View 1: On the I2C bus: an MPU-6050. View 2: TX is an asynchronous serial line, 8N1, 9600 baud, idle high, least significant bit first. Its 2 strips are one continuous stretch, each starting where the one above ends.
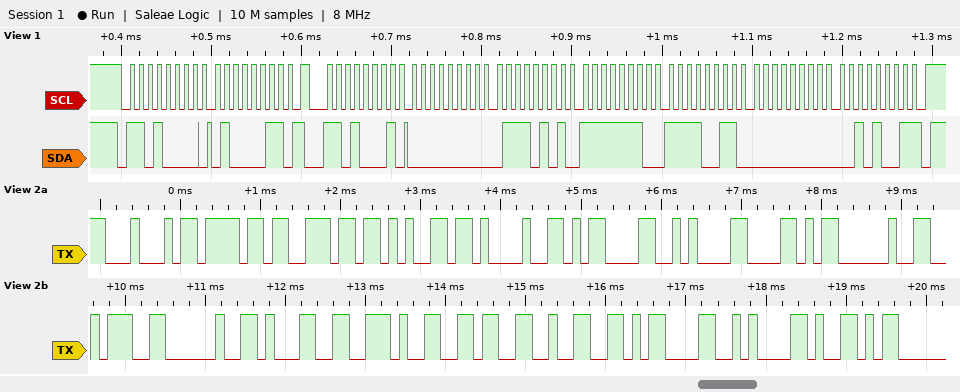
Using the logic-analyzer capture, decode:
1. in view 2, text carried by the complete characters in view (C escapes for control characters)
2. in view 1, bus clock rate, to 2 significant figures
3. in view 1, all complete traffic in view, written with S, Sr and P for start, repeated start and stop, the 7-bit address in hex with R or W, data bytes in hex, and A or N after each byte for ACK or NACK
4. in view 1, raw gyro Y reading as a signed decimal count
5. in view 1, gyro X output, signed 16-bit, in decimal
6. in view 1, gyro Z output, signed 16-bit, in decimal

"Done!\r\nX : 1.62\r\nY"
100 kHz
S 68W A 43 A Sr 68R A 00 A 75 A FE A F3 A 00 A 29 N P
-269
117
41
